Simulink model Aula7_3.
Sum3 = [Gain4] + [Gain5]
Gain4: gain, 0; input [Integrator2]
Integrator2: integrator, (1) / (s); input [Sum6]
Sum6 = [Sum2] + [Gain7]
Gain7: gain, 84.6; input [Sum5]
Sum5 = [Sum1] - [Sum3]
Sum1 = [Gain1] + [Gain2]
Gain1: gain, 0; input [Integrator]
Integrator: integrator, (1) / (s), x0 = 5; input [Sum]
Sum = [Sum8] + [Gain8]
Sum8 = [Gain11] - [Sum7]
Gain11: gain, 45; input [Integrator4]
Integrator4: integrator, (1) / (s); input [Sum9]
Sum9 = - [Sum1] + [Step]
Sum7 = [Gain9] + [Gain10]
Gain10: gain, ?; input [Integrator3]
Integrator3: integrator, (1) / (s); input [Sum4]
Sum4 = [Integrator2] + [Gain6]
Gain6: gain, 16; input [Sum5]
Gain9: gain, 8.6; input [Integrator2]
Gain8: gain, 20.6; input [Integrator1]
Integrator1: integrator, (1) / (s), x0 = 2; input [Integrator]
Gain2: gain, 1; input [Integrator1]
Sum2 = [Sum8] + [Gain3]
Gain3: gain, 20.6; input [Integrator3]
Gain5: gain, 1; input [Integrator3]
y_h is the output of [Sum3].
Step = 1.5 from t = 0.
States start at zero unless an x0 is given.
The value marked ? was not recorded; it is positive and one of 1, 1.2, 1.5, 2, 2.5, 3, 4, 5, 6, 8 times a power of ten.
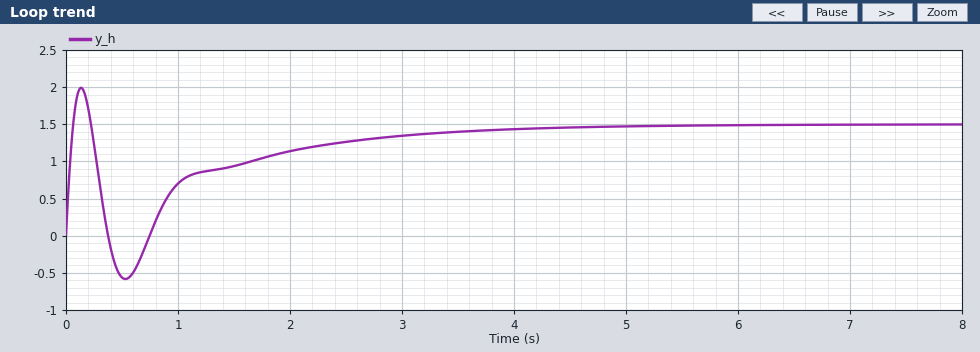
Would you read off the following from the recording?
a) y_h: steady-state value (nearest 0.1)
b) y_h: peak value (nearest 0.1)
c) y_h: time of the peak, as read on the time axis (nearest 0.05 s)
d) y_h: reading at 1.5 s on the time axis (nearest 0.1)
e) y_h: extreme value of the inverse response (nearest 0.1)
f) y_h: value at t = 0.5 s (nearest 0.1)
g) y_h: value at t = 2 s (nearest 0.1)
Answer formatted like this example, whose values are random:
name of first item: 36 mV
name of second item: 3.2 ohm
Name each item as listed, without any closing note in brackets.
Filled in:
y_h: steady-state value: 1.5
y_h: peak value: 2.0
y_h: time of the peak, as read on the time axis: 0.15 s
y_h: reading at 1.5 s on the time axis: 0.9
y_h: extreme value of the inverse response: -0.6
y_h: value at t = 0.5 s: -0.6
y_h: value at t = 2 s: 1.1
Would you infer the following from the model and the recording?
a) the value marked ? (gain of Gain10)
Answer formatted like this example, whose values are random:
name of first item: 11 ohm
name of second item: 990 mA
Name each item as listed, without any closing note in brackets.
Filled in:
the value marked ?: 80
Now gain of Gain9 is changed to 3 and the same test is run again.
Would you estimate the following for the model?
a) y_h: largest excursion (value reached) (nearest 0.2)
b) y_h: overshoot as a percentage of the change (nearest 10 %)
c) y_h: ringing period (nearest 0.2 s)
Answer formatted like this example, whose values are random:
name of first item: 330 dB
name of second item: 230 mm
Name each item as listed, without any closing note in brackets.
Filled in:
y_h: largest excursion (value reached): 2.0
y_h: overshoot as a percentage of the change: 40 %
y_h: ringing period: 0.8 s
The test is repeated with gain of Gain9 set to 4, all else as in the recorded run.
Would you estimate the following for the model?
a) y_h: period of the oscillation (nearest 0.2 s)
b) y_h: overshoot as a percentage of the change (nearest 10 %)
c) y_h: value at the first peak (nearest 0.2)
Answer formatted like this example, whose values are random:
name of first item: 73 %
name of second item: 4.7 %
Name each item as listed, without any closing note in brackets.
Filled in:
y_h: period of the oscillation: 0.8 s
y_h: overshoot as a percentage of the change: 40 %
y_h: value at the first peak: 2.0
